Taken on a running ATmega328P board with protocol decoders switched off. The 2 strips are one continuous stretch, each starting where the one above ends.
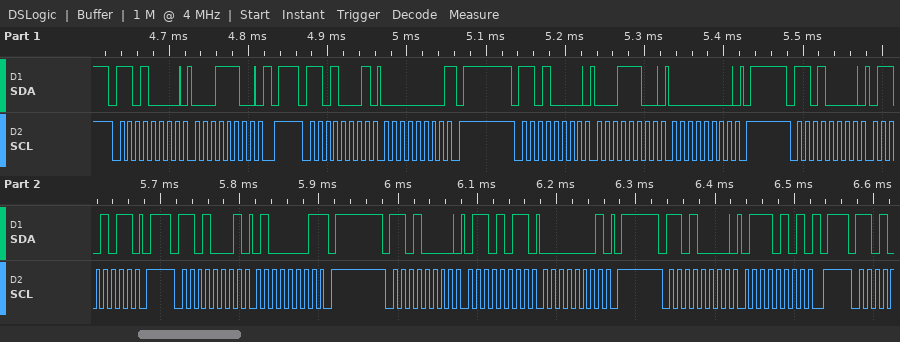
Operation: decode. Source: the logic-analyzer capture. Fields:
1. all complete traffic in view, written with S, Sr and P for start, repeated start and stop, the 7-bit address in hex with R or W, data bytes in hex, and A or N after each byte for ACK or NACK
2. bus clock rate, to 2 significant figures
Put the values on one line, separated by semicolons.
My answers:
S 68W A 1C A P S 68R A 00 N P S 68W A 1C A 00 A P S 68W A 6B A P S 68R A 41 N P S 68W A 6B A 01 A P S 68W A 75 A P; 100 kHz
